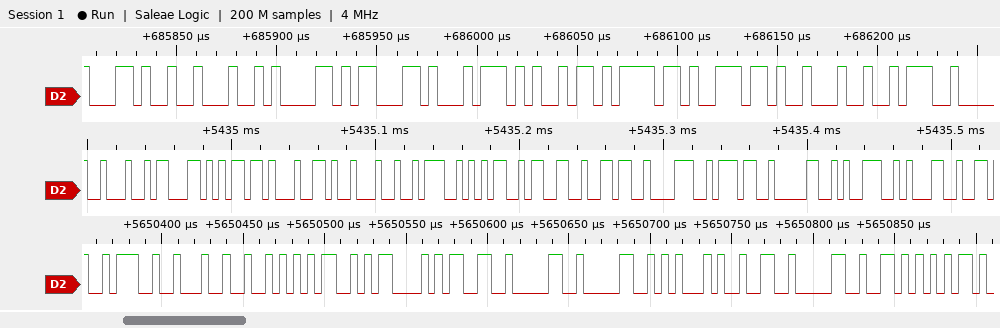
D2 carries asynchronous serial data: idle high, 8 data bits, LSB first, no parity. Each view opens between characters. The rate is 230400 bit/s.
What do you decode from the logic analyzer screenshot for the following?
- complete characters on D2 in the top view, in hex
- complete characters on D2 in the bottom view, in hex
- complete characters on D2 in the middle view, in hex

2C, 22, 61, 63, 74, 69, 6F, 6E, 22, 3A
3A, 22, 52, 4D, 43, 33, 30, 30, 45, 32, 30, 56
22, 63, 6D, 64, 22, 3A, 35, 33, 36, 38, 37, 30, 39, 31
